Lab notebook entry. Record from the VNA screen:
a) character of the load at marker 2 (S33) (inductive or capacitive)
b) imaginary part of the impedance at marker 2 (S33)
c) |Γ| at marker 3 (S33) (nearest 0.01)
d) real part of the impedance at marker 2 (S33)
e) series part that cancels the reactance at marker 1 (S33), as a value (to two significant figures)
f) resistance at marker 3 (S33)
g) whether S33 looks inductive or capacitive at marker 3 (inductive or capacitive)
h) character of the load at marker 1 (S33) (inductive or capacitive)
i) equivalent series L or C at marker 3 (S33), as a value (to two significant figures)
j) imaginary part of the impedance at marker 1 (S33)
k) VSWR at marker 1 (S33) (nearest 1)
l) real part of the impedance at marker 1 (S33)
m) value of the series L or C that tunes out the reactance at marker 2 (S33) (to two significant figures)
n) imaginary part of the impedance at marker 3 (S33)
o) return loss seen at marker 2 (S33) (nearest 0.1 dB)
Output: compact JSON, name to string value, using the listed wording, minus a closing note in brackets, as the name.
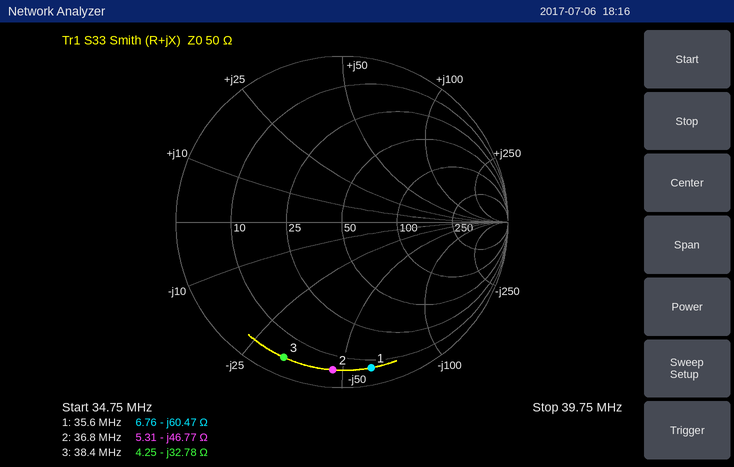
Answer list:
{"character of the load at marker 2 (S33)": "capacitive", "imaginary part of the impedance at marker 2": "-46.77 Ω", "|Γ| at marker 3 (S33)": "0.89", "real part of the impedance at marker 2": "5.31 Ω", "series part that cancels the reactance at marker 1 (S33), as a value": "270 nH", "resistance at marker 3": "4.25 Ω", "whether S33 looks inductive or capacitive at marker 3": "capacitive", "character of the load at marker 1 (S33)": "capacitive", "equivalent series L or C at marker 3 (S33), as a value": "130 pF", "imaginary part of the impedance at marker 1": "-60.47 Ω", "VSWR at marker 1 (S33)": "18", "real part of the impedance at marker 1": "6.76 Ω", "value of the series L or C that tunes out the reactance at marker 2 (S33)": "200 nH", "imaginary part of the impedance at marker 3": "-32.78 Ω", "return loss seen at marker 2 (S33)": "1.0 dB"}
